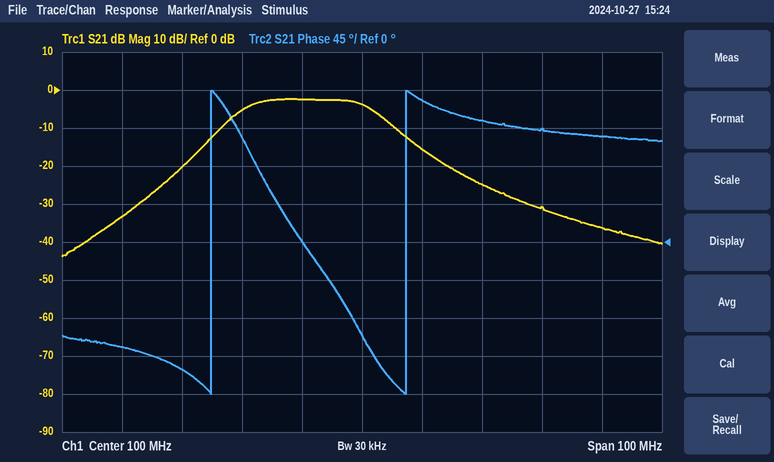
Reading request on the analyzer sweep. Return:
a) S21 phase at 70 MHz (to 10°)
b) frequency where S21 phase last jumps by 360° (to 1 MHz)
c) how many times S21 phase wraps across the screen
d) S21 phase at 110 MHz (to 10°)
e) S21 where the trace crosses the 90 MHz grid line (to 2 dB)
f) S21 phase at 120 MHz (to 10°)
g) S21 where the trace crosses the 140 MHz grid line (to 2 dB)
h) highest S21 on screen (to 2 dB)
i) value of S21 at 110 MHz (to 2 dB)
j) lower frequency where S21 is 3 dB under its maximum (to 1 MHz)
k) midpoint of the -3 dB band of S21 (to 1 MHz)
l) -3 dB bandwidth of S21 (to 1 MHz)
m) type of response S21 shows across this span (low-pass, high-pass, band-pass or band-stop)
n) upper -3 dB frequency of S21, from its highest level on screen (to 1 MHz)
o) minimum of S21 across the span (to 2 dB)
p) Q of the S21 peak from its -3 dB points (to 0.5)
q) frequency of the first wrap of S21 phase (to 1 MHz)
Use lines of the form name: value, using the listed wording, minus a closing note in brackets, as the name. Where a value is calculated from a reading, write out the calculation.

S21 phase at 70 MHz: -150°
frequency where S21 phase last jumps by 360°: 107 MHz
how many times S21 phase wraps across the screen: 2
S21 phase at 110 MHz: 170°
S21 where the trace crosses the 90 MHz grid line: -2 dB
S21 phase at 120 MHz: 140°
S21 where the trace crosses the 140 MHz grid line: -36 dB
highest S21 on screen: -2 dB
value of S21 at 110 MHz: -16 dB
lower frequency where S21 is 3 dB under its maximum: 80 MHz
midpoint of the -3 dB band of S21: 91 MHz
-3 dB bandwidth of S21: 102 MHz − 80 MHz = 22 MHz
type of response S21 shows across this span: band-pass
upper -3 dB frequency of S21, from its highest level on screen: 102 MHz
minimum of S21 across the span: -44 dB
Q of the S21 peak from its -3 dB points: 91 MHz / 22 MHz ≈ 4.14, so 4.0 to the nearest 0.5
frequency of the first wrap of S21 phase: 75 MHz
